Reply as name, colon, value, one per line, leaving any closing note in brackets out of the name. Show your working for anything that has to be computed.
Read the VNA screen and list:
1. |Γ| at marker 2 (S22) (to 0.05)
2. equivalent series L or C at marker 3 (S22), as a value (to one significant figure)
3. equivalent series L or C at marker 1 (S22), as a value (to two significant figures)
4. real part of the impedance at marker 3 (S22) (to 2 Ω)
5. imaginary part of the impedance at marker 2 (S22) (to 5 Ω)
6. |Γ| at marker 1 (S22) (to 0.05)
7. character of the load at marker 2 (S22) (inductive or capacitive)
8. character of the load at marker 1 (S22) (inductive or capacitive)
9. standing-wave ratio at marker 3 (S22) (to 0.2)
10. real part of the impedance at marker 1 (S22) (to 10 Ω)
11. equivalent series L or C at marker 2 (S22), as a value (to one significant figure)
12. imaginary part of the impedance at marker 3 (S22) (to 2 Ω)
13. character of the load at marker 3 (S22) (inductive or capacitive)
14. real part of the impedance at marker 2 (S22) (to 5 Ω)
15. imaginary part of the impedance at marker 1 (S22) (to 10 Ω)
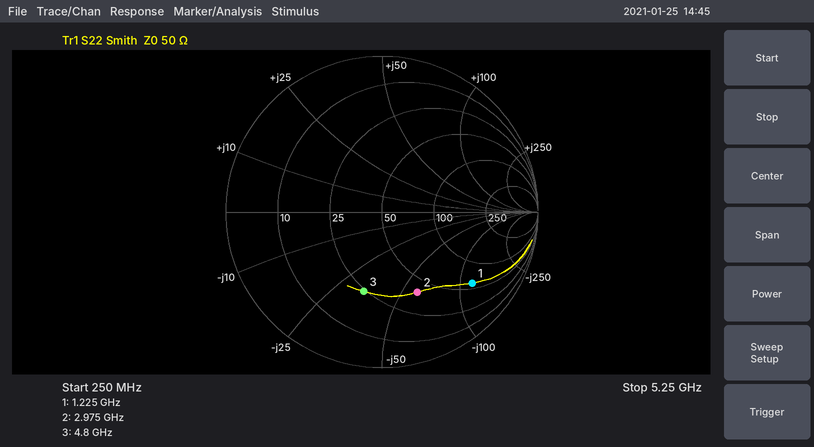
|Γ| at marker 2 (S22): 0.55
equivalent series L or C at marker 3 (S22), as a value: C = 1/(2π × 4.8 GHz × 34 Ω) ≈ 1.0 pF
equivalent series L or C at marker 1 (S22), as a value: C = 1/(2π × 1.225 GHz × 120 Ω) ≈ 1.1 pF
real part of the impedance at marker 3 (S22): 24 Ω
imaginary part of the impedance at marker 2 (S22): -60 Ω
|Γ| at marker 1 (S22): 0.75
character of the load at marker 2 (S22): capacitive
character of the load at marker 1 (S22): capacitive
standing-wave ratio at marker 3 (S22): 3.2
real part of the impedance at marker 1 (S22): 60 Ω
equivalent series L or C at marker 2 (S22), as a value: C = 1/(2π × 2.975 GHz × 60 Ω) ≈ 892 fF, so 900 fF to one significant figure
imaginary part of the impedance at marker 3 (S22): -34 Ω
character of the load at marker 3 (S22): capacitive
real part of the impedance at marker 2 (S22): 40 Ω
imaginary part of the impedance at marker 1 (S22): -120 Ω
